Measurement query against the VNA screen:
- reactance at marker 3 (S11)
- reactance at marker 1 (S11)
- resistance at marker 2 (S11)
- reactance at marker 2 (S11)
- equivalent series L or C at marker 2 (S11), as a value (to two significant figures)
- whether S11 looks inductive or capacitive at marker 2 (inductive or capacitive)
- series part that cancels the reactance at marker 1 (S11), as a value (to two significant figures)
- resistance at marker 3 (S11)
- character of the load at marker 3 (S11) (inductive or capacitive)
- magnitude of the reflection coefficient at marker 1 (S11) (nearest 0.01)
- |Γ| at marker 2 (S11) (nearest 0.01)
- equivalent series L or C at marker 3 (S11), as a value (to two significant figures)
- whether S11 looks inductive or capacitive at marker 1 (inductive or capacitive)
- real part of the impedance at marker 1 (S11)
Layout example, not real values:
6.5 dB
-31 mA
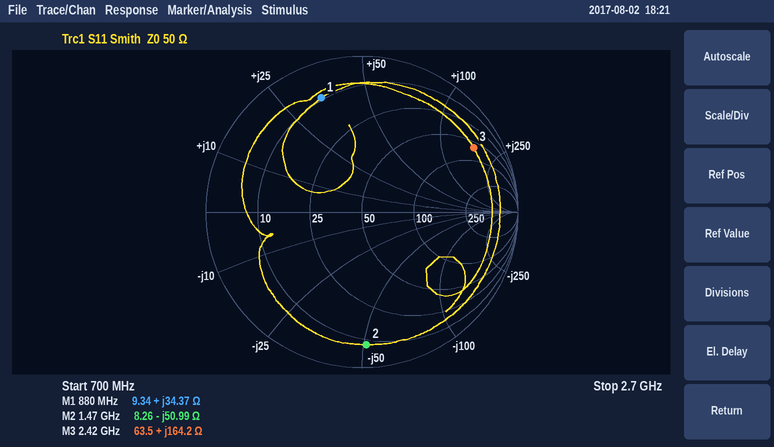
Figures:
+164.2 Ω
+34.37 Ω
8.26 Ω
-50.99 Ω
2.1 pF
capacitive
5.3 pF
63.5 Ω
inductive
0.78
0.85
11 nH
inductive
9.34 Ω
